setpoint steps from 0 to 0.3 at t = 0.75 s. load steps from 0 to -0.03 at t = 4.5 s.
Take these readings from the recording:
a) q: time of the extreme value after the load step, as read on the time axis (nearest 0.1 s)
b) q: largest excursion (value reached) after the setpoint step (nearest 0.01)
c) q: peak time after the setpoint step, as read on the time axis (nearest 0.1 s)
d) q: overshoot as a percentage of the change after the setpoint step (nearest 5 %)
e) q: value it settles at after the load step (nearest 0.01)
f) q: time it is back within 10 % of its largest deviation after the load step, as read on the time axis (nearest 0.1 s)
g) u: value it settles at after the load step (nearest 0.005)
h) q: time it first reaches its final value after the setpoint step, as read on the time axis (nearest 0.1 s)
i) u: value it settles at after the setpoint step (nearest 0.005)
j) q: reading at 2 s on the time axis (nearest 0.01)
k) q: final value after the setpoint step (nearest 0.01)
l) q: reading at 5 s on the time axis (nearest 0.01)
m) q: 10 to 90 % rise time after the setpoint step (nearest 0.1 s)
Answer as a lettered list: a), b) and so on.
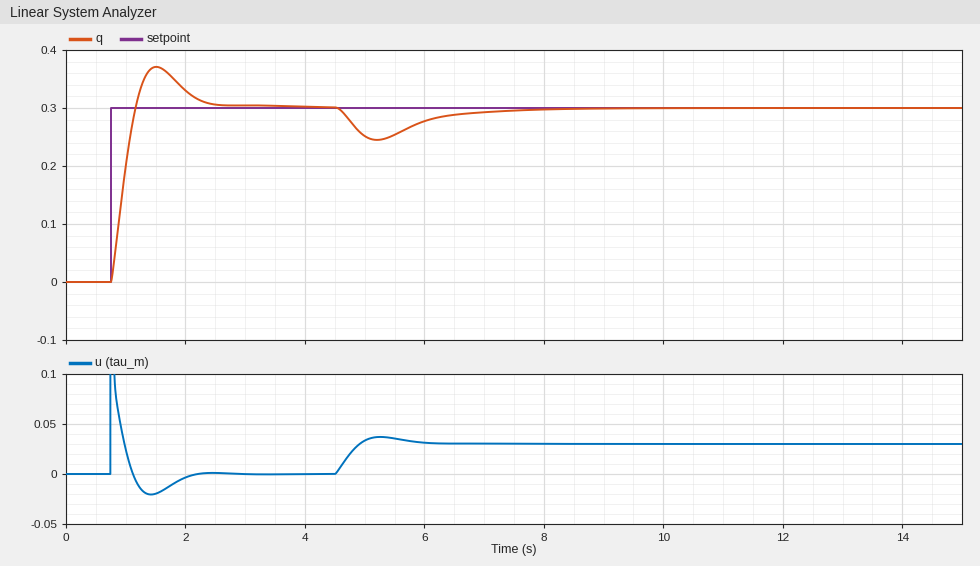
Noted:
a) 5.2 s
b) 0.37
c) 1.5 s
d) 25 %
e) 0.30
f) 7.3 s
g) 0.030
h) 1.2 s
i) 0.000
j) 0.33
k) 0.30
l) 0.25
m) 0.3 s
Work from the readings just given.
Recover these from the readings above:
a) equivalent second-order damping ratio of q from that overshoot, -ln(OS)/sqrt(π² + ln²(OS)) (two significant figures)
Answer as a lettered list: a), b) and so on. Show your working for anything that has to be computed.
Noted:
a) ln(0.25) = -1.386; 1.386 / sqrt(9.870 + 1.922) = 0.40
